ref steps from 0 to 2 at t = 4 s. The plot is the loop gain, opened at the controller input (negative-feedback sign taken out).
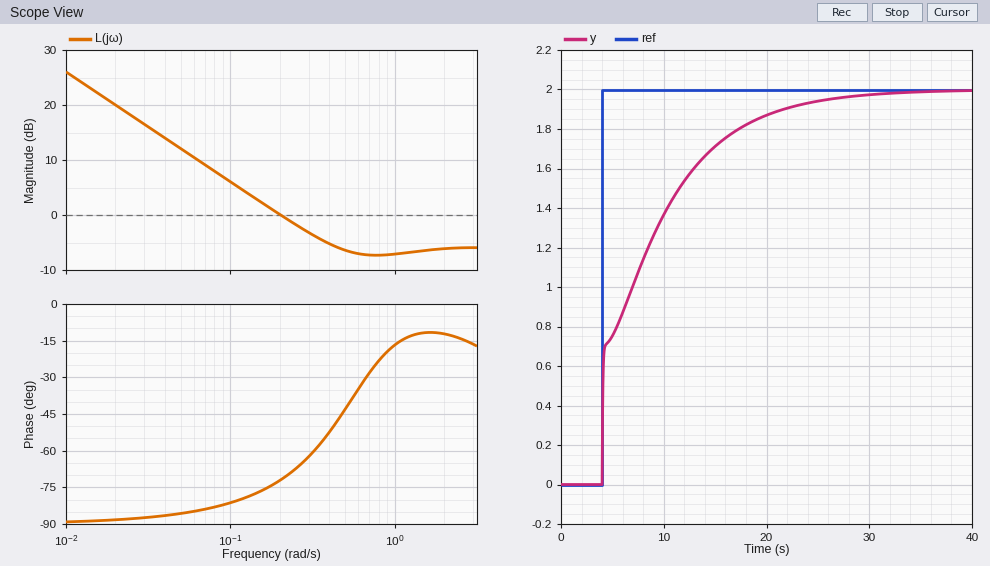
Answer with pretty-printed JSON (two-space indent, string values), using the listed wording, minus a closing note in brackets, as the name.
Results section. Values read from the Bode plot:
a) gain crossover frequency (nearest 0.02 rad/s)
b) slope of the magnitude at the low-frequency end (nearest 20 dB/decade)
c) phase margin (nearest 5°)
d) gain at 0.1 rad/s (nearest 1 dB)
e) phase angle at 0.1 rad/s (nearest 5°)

{
  "gain crossover frequency": "0.20 rad/s",
  "slope of the magnitude at the low-frequency end": "-20 dB/decade",
  "phase margin": "110°",
  "gain at 0.1 rad/s": "6 dB",
  "phase angle at 0.1 rad/s": "-80°"
}
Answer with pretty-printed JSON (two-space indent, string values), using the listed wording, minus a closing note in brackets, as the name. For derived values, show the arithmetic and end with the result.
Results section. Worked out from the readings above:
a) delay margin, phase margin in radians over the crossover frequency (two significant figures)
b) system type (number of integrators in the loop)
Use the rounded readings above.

{
  "delay margin, phase margin in radians over the crossover frequency": "110 × π / 180 / 0.2 = 9.6 s",
  "system type": "1"
}
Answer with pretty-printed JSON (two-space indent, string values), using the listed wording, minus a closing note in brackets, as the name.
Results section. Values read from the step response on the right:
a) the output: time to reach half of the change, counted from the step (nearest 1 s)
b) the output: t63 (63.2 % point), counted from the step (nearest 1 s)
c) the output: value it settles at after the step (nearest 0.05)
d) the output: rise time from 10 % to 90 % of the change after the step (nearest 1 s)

{
  "the output: time to reach half of the change, counted from the step": "3 s",
  "the output: t63 (63.2 % point), counted from the step": "5 s",
  "the output: value it settles at after the step": "2.00",
  "the output: rise time from 10 % to 90 % of the change after the step": "13 s"
}
